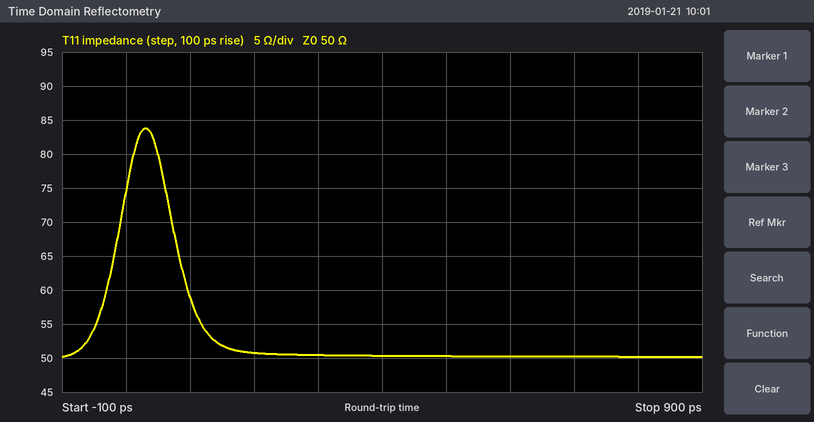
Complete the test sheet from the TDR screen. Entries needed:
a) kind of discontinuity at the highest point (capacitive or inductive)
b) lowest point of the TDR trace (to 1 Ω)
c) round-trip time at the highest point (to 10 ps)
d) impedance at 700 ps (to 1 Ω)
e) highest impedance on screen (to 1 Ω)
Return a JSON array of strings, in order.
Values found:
["inductive", "50 Ω", "30 ps", "50 Ω", "84 Ω"]
